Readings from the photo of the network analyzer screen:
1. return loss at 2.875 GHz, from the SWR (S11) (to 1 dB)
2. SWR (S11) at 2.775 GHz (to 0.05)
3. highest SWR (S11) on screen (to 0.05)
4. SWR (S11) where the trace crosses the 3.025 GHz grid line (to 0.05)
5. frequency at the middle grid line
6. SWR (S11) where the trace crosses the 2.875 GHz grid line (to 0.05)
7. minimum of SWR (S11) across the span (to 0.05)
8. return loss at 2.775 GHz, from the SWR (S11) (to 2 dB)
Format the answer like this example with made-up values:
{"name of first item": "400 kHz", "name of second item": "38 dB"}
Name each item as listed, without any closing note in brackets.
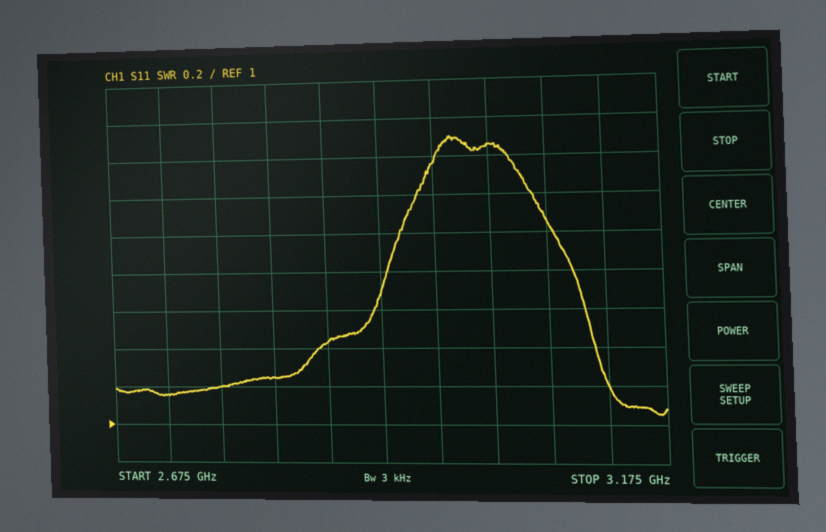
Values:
{"return loss at 2.875 GHz, from the SWR (S11)": "15 dB", "SWR (S11) at 2.775 GHz": "1.20", "highest SWR (S11) on screen": "2.50", "SWR (S11) where the trace crosses the 3.025 GHz grid line": "2.45", "frequency at the middle grid line": "2.925 GHz", "SWR (S11) where the trace crosses the 2.875 GHz grid line": "1.45", "minimum of SWR (S11) across the span": "1.05", "return loss at 2.775 GHz, from the SWR (S11)": "20 dB"}
